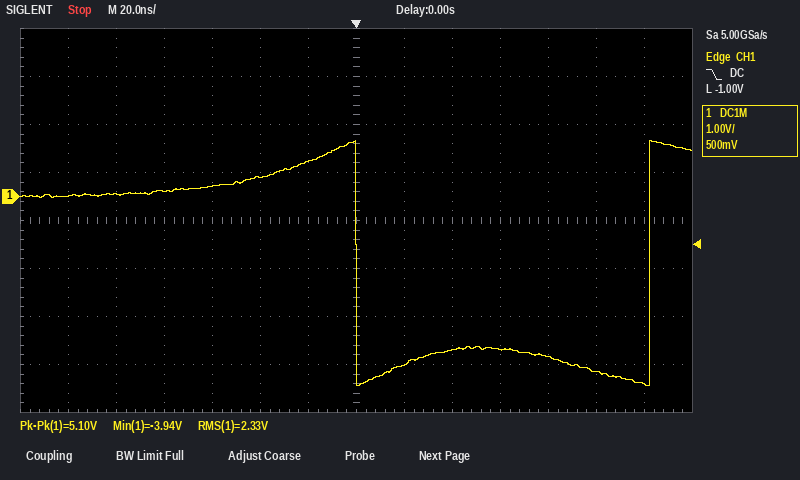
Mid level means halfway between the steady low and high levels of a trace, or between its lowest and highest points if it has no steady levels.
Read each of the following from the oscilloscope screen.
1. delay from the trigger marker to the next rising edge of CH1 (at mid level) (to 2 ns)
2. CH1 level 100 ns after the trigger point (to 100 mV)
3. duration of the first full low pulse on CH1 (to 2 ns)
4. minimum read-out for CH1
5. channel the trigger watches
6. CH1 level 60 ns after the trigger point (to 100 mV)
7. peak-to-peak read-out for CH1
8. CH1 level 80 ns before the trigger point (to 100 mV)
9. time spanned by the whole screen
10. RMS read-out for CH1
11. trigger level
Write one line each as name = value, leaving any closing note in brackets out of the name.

delay from the trigger marker to the next rising edge of CH1 (at mid level) = 122 ns
CH1 level 100 ns after the trigger point = -3.6 V
duration of the first full low pulse on CH1 = 122 ns
minimum read-out for CH1 = -3.94 V
channel the trigger watches = CH1
CH1 level 60 ns after the trigger point = -3.2 V
peak-to-peak read-out for CH1 = 5.10 V
CH1 level 80 ns before the trigger point = 100 mV
time spanned by the whole screen = 280 ns
RMS read-out for CH1 = 2.33 V
trigger level = -1.00 V
